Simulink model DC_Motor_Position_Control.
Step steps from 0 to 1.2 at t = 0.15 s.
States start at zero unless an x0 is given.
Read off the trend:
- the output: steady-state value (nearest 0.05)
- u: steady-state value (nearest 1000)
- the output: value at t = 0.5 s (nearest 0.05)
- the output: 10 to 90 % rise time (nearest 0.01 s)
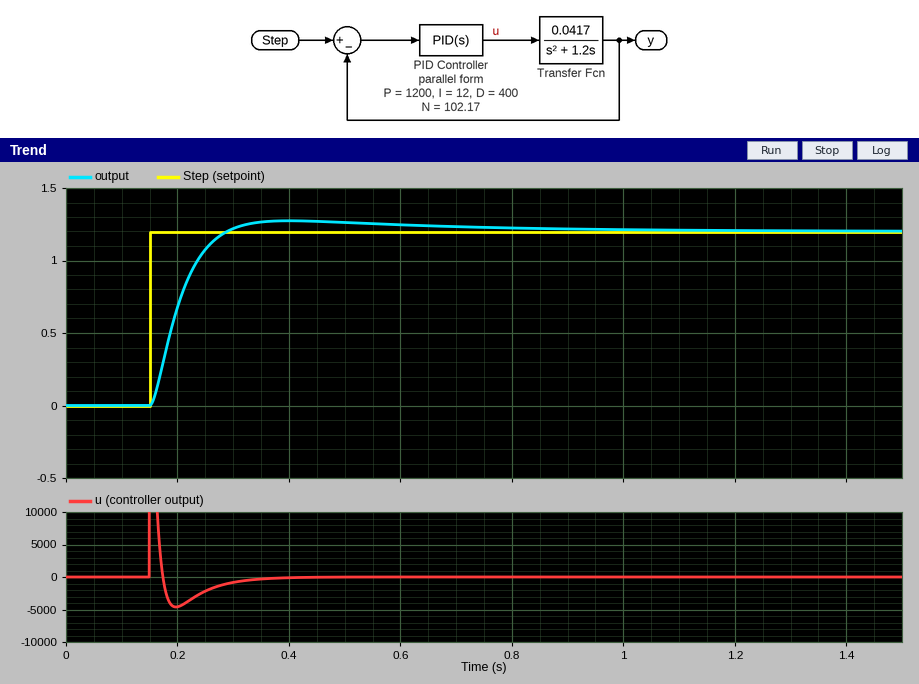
1.20
0
1.25
0.09 s
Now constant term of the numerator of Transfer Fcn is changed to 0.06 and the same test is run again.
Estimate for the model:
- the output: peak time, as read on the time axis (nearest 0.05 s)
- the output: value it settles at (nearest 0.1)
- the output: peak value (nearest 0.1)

0.30 s
1.2
1.3
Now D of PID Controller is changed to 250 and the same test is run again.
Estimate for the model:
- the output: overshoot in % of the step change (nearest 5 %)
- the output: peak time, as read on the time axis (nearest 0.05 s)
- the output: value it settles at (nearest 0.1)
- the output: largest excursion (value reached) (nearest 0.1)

15 %
0.45 s
1.2
1.4
